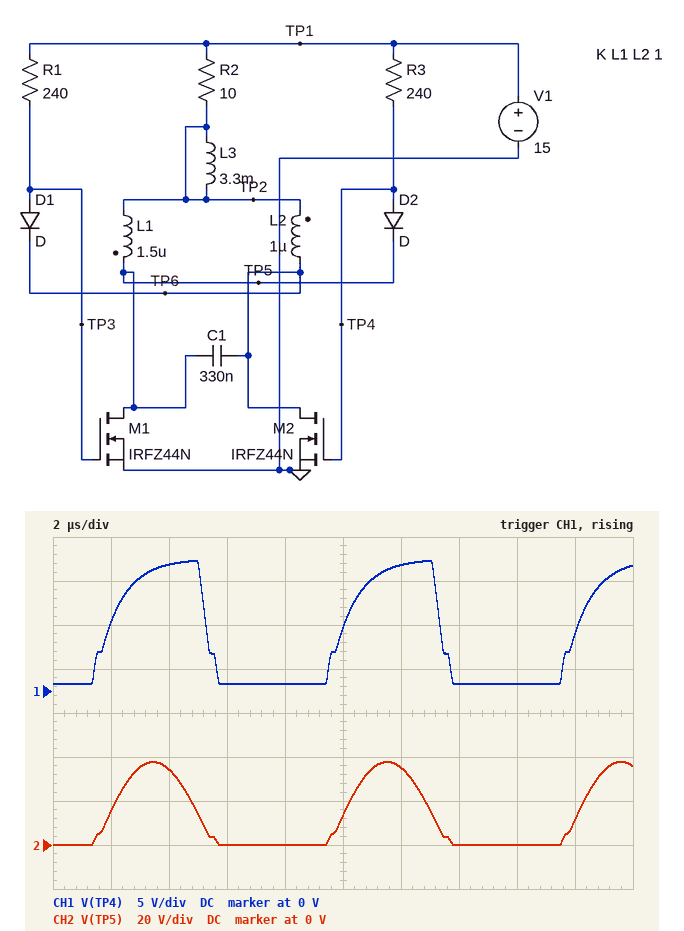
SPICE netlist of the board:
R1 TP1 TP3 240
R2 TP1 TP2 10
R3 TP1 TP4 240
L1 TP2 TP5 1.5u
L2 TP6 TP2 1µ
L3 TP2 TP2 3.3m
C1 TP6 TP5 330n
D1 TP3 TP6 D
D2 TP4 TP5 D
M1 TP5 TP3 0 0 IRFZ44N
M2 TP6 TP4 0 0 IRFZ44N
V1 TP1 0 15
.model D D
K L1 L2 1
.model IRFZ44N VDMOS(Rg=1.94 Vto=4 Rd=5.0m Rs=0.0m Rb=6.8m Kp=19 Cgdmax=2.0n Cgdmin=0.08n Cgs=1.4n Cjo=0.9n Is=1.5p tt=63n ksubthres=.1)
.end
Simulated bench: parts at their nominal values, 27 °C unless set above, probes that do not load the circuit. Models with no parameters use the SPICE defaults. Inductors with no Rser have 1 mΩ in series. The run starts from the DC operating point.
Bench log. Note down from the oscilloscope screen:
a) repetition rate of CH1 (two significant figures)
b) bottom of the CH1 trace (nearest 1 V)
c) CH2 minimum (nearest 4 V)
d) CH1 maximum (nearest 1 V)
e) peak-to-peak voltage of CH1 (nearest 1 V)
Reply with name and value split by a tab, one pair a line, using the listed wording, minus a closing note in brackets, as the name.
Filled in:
repetition rate of CH1	120 kHz
bottom of the CH1 trace	1 V
CH2 minimum	0 V
CH1 maximum	15 V
peak-to-peak voltage of CH1	14 V
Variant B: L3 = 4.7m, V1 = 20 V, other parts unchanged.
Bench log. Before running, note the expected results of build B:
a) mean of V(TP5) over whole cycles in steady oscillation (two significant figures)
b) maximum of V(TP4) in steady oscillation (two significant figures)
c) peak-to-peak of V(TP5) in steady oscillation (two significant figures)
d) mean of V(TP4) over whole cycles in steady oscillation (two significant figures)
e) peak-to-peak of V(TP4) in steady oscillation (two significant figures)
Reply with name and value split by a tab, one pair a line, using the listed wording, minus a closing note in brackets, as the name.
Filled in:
mean of V(TP5) over whole cycles in steady oscillation	16 V
maximum of V(TP4) in steady oscillation	20 V
peak-to-peak of V(TP5) in steady oscillation	50 V
mean of V(TP4) over whole cycles in steady oscillation	8.0 V
peak-to-peak of V(TP4) in steady oscillation	19 V
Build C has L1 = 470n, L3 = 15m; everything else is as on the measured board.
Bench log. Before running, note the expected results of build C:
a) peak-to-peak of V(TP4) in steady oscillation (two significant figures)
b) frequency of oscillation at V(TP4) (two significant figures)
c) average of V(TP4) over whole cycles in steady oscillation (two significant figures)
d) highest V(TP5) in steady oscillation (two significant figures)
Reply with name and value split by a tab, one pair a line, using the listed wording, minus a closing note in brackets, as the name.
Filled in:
peak-to-peak of V(TP4) in steady oscillation	14 V
frequency of oscillation at V(TP4)	160 kHz
average of V(TP4) over whole cycles in steady oscillation	5.8 V
highest V(TP5) in steady oscillation	37 V
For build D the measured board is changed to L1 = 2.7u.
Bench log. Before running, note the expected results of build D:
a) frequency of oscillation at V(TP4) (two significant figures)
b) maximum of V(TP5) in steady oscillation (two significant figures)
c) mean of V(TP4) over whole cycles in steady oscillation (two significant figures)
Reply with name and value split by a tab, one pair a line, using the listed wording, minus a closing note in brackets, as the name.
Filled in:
frequency of oscillation at V(TP4)	100 kHz
maximum of V(TP5) in steady oscillation	36 V
mean of V(TP4) over whole cycles in steady oscillation	6.4 V
